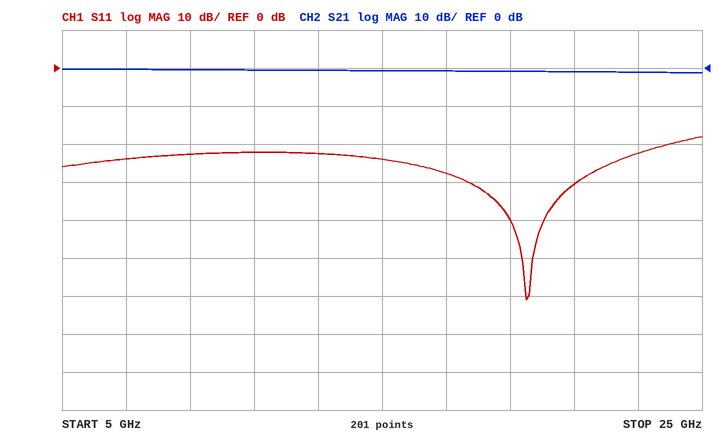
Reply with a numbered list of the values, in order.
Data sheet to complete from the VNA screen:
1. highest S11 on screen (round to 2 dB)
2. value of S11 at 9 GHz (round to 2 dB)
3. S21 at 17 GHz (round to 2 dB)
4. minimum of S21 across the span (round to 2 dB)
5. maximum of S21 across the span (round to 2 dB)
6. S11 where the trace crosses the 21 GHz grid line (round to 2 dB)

1. -18 dB
2. -22 dB
3. 0 dB
4. -2 dB
5. 0 dB
6. -30 dB
